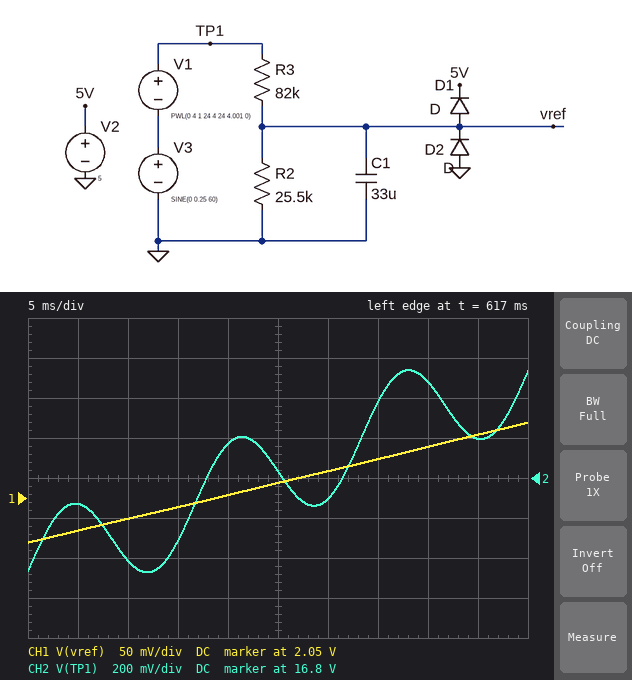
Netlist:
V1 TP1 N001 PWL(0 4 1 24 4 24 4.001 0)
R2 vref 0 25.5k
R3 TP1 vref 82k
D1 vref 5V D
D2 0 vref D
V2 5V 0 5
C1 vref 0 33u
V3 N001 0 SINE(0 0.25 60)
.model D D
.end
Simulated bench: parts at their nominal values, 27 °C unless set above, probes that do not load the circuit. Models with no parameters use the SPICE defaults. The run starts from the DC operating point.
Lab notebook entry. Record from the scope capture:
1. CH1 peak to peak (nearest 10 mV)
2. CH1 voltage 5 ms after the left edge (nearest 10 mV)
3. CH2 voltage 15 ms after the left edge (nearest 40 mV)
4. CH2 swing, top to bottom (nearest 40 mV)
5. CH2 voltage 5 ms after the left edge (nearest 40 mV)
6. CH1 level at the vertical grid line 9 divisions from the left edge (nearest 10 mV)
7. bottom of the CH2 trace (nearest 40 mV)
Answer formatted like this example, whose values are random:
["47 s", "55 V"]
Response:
["150 mV", "2.01 V", "16.48 V", "1.00 V", "16.68 V", "2.13 V", "16.32 V"]
